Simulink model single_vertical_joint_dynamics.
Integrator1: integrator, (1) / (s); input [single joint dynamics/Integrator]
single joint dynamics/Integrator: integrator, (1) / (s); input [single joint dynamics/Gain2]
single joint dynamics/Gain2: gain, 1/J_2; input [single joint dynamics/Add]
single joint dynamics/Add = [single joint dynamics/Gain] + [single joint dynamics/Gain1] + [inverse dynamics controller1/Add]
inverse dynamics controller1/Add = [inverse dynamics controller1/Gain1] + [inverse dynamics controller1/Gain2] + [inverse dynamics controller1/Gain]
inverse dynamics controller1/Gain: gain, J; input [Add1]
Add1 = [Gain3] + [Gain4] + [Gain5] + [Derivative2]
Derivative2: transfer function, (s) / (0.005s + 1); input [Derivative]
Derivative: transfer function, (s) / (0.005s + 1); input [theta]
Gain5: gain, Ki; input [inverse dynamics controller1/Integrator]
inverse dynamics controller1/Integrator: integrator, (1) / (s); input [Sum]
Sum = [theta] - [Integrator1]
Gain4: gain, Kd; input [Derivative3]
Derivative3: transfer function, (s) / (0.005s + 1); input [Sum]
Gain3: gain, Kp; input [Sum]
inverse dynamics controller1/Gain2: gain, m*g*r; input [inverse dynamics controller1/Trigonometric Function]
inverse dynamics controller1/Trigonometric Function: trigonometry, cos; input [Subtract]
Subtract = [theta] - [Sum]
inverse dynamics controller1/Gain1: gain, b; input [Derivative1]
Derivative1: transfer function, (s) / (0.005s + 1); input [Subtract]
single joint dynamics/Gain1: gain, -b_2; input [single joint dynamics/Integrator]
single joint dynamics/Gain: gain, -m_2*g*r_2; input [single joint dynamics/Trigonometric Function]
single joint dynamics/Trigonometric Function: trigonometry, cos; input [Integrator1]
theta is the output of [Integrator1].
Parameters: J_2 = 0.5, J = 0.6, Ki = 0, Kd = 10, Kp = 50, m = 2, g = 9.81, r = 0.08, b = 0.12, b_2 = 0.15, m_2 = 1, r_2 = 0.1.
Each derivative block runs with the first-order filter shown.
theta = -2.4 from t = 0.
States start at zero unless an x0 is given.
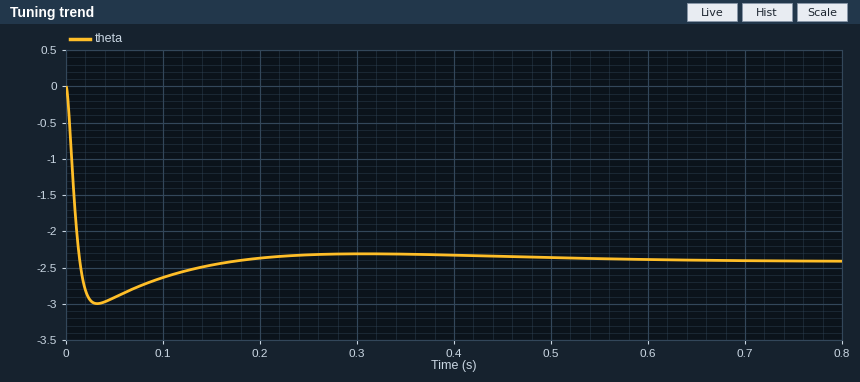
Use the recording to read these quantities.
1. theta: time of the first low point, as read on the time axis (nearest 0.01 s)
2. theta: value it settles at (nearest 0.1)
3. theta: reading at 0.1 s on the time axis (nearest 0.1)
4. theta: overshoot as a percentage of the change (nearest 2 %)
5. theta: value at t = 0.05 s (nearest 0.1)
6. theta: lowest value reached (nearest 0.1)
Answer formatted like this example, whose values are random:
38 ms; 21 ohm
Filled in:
0.03 s; -2.4; -2.6; 24 %; -2.9; -3.0
